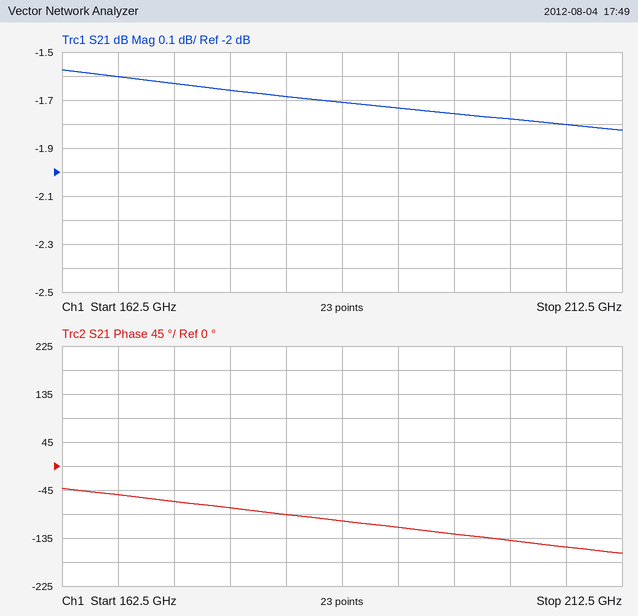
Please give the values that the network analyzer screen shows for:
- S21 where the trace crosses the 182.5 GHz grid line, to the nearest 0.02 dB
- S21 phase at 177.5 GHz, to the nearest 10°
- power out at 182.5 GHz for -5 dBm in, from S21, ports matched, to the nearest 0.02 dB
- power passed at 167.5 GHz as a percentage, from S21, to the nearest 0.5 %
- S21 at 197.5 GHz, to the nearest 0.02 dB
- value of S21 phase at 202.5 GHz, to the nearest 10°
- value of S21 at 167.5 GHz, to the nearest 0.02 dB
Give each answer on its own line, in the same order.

-1.68 dB
-80°
-6.68 dBm
69.0 %
-1.76 dB
-140°
-1.60 dB
